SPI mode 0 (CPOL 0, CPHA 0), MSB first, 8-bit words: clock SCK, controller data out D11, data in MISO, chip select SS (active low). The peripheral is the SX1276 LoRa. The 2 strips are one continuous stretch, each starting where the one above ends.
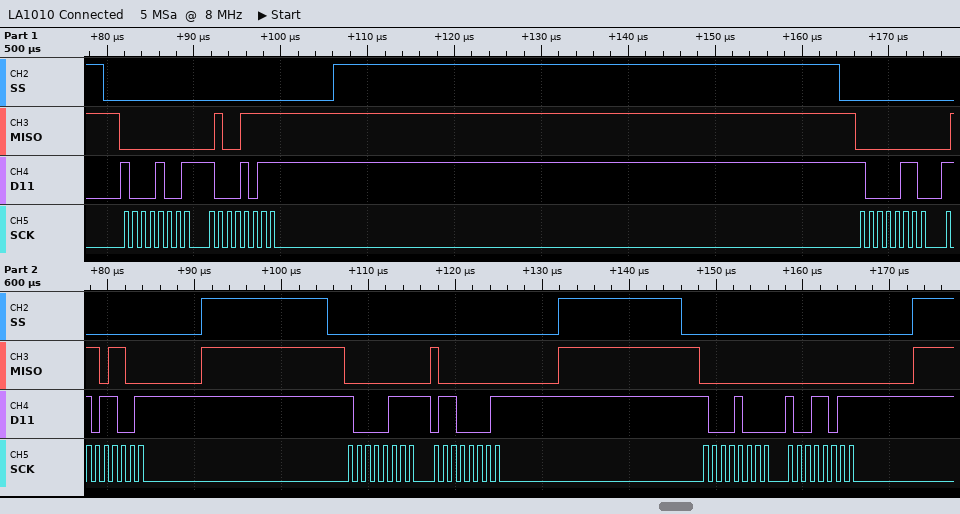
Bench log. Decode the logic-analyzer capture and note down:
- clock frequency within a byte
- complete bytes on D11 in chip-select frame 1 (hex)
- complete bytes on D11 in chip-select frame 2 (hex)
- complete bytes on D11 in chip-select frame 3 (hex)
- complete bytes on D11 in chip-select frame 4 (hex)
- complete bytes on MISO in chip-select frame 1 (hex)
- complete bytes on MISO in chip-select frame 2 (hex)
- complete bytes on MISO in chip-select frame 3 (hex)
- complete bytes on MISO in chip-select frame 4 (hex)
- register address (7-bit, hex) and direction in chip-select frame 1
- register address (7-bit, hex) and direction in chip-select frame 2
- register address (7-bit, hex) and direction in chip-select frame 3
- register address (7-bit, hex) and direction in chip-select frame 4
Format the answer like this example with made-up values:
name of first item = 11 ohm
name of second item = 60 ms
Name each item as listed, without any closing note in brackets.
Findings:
clock frequency within a byte = 1 MHz
complete bytes on D11 in chip-select frame 1 = 89 8B
complete bytes on D11 in chip-select frame 2 = 86 D9
complete bytes on D11 in chip-select frame 3 = 87 61
complete bytes on D11 in chip-select frame 4 = 88 9B
complete bytes on MISO in chip-select frame 1 = 00 4F
complete bytes on MISO in chip-select frame 2 = 00 6C
complete bytes on MISO in chip-select frame 3 = 00 80
complete bytes on MISO in chip-select frame 4 = 00 00
register address (7-bit, hex) and direction in chip-select frame 1 = 0x09 write
register address (7-bit, hex) and direction in chip-select frame 2 = 0x06 write
register address (7-bit, hex) and direction in chip-select frame 3 = 0x07 write
register address (7-bit, hex) and direction in chip-select frame 4 = 0x08 write
